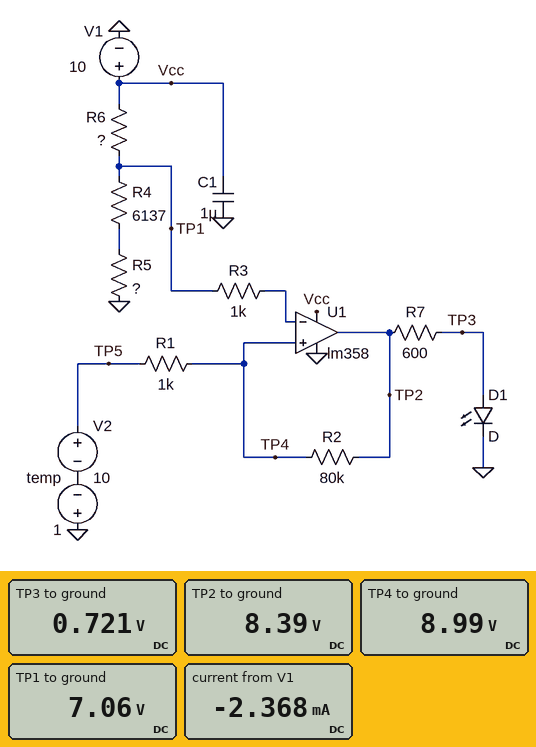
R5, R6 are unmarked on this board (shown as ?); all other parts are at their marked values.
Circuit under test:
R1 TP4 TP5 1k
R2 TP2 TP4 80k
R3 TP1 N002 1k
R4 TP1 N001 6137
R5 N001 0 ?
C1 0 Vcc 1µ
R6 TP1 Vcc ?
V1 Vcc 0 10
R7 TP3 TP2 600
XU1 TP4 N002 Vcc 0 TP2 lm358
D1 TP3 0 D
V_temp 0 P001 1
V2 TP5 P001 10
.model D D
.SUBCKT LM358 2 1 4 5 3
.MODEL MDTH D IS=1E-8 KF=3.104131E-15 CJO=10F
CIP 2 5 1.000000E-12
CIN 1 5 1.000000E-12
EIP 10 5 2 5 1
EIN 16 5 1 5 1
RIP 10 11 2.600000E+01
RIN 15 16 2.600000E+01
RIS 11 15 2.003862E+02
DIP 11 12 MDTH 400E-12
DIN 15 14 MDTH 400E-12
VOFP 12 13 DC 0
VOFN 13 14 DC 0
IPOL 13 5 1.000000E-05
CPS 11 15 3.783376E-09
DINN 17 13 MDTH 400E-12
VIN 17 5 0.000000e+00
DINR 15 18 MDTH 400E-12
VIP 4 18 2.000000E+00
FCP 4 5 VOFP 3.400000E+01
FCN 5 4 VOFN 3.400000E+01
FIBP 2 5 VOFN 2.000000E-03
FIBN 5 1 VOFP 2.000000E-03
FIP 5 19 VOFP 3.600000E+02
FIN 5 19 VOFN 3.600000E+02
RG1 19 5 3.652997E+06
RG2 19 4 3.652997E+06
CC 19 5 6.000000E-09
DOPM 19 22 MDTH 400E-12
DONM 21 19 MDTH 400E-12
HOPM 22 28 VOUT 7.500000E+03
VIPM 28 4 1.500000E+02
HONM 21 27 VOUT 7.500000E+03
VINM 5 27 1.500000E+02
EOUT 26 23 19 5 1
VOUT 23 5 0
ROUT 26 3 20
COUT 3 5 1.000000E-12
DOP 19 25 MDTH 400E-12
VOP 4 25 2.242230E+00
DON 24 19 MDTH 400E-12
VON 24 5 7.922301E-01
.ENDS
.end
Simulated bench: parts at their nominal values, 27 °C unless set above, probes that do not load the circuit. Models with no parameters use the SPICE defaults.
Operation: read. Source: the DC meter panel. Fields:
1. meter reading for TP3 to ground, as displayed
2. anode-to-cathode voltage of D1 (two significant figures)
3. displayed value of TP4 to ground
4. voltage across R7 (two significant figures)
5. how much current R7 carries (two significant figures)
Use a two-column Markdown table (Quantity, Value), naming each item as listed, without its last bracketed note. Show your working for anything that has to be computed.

| Quantity | Value |
|---|---|
| meter reading for TP3 to ground, as displayed | 0.721 V |
| anode-to-cathode voltage of D1 | 721 mV = 720 mV |
| displayed value of TP4 to ground | 8.99 V |
| voltage across R7 | 8.39 V - 721 mV = 7.7 V |
| how much current R7 carries | (8.39 V - 721 mV) / 600 Ω = 13 mA |
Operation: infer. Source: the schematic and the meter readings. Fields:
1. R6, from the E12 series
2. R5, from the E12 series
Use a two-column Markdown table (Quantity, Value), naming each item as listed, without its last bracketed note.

| Quantity | Value |
|---|---|
| R6, from the E12 series | 3.3 kΩ |
| R5, from the E12 series | 1.8 kΩ |
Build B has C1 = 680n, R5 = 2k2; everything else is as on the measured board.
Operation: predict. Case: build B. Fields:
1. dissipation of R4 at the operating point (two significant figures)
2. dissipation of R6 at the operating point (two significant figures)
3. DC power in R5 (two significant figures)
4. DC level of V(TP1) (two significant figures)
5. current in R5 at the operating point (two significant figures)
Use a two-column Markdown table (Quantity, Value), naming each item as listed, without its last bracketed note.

| Quantity | Value |
|---|---|
| dissipation of R4 at the operating point | 4.5 mW |
| dissipation of R6 at the operating point | 2.4 mW |
| DC power in R5 | 1.6 mW |
| DC level of V(TP1) | 7.2 V |
| current in R5 at the operating point | 860 µA |
